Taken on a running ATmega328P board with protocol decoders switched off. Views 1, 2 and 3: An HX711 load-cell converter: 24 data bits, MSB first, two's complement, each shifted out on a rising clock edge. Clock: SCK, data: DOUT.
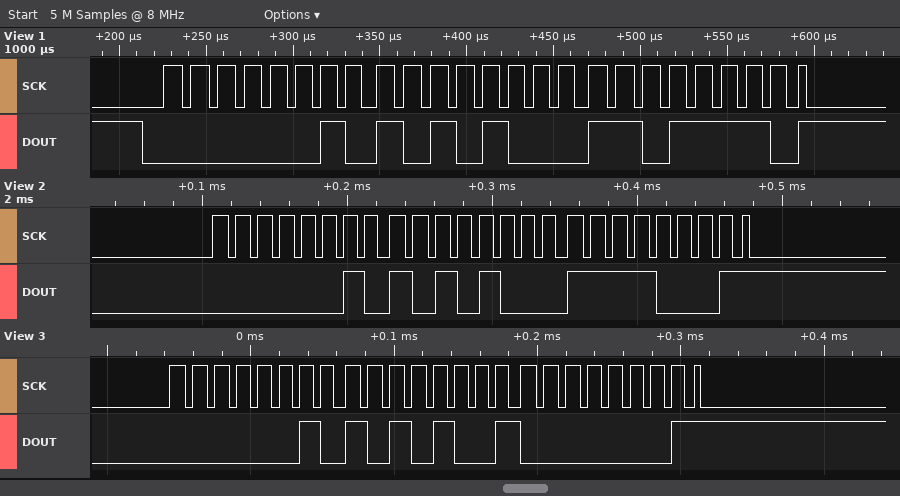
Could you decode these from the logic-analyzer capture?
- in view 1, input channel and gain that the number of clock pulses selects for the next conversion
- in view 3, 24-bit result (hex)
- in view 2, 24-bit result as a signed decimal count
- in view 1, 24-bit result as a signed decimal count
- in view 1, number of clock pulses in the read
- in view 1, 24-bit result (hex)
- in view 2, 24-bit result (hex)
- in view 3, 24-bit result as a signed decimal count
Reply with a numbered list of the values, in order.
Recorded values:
1. channel A, gain 128
2. 0x02A901
3. 174321
4. 174302
5. 25
6. 0x02A8DE
7. 0x02A8F1
8. 174337
